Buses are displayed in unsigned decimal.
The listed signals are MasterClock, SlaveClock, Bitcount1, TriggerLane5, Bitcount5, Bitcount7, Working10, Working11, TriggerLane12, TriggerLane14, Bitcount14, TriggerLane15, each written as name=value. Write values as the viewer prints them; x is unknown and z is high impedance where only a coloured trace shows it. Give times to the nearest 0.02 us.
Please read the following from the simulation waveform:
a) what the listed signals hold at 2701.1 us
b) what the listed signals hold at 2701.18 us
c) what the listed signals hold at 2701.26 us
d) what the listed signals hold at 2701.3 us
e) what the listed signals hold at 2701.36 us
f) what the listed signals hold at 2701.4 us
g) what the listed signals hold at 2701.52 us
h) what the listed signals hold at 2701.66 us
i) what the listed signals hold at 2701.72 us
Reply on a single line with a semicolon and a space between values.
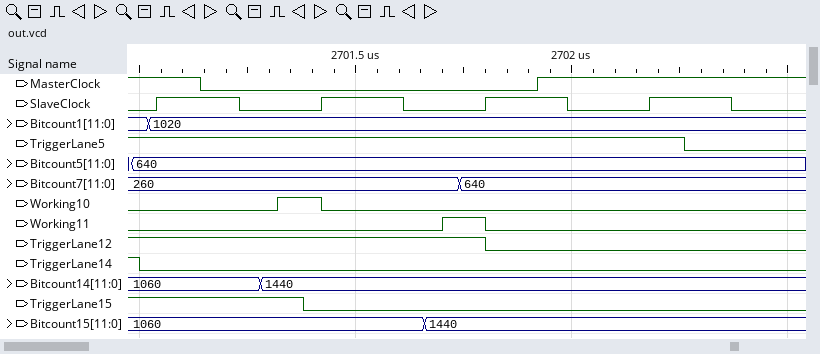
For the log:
MasterClock=1, SlaveClock=1, Bitcount1=1020, TriggerLane5=1, Bitcount5=640, Bitcount7=260, Working10=0, Working11=0, TriggerLane12=1, TriggerLane14=0, Bitcount14=1060, TriggerLane15=1; MasterClock=0, SlaveClock=1, Bitcount1=1020, TriggerLane5=1, Bitcount5=640, Bitcount7=260, Working10=0, Working11=0, TriggerLane12=1, TriggerLane14=0, Bitcount14=1060, TriggerLane15=1; MasterClock=0, SlaveClock=0, Bitcount1=1020, TriggerLane5=1, Bitcount5=640, Bitcount7=260, Working10=0, Working11=0, TriggerLane12=1, TriggerLane14=0, Bitcount14=1060, TriggerLane15=1; MasterClock=0, SlaveClock=0, Bitcount1=1020, TriggerLane5=1, Bitcount5=640, Bitcount7=260, Working10=0, Working11=0, TriggerLane12=1, TriggerLane14=0, Bitcount14=1440, TriggerLane15=1; MasterClock=0, SlaveClock=0, Bitcount1=1020, TriggerLane5=1, Bitcount5=640, Bitcount7=260, Working10=1, Working11=0, TriggerLane12=1, TriggerLane14=0, Bitcount14=1440, TriggerLane15=1; MasterClock=0, SlaveClock=0, Bitcount1=1020, TriggerLane5=1, Bitcount5=640, Bitcount7=260, Working10=1, Working11=0, TriggerLane12=1, TriggerLane14=0, Bitcount14=1440, TriggerLane15=0; MasterClock=0, SlaveClock=1, Bitcount1=1020, TriggerLane5=1, Bitcount5=640, Bitcount7=260, Working10=0, Working11=0, TriggerLane12=1, TriggerLane14=0, Bitcount14=1440, TriggerLane15=0; MasterClock=0, SlaveClock=0, Bitcount1=1020, TriggerLane5=1, Bitcount5=640, Bitcount7=260, Working10=0, Working11=0, TriggerLane12=1, TriggerLane14=0, Bitcount14=1440, TriggerLane15=0; MasterClock=0, SlaveClock=0, Bitcount1=1020, TriggerLane5=1, Bitcount5=640, Bitcount7=260, Working10=0, Working11=1, TriggerLane12=1, TriggerLane14=0, Bitcount14=1440, TriggerLane15=0
